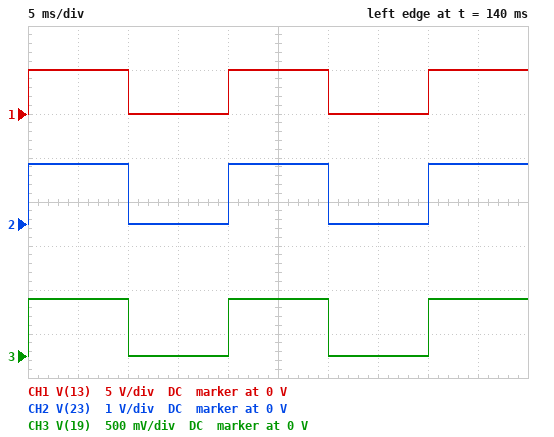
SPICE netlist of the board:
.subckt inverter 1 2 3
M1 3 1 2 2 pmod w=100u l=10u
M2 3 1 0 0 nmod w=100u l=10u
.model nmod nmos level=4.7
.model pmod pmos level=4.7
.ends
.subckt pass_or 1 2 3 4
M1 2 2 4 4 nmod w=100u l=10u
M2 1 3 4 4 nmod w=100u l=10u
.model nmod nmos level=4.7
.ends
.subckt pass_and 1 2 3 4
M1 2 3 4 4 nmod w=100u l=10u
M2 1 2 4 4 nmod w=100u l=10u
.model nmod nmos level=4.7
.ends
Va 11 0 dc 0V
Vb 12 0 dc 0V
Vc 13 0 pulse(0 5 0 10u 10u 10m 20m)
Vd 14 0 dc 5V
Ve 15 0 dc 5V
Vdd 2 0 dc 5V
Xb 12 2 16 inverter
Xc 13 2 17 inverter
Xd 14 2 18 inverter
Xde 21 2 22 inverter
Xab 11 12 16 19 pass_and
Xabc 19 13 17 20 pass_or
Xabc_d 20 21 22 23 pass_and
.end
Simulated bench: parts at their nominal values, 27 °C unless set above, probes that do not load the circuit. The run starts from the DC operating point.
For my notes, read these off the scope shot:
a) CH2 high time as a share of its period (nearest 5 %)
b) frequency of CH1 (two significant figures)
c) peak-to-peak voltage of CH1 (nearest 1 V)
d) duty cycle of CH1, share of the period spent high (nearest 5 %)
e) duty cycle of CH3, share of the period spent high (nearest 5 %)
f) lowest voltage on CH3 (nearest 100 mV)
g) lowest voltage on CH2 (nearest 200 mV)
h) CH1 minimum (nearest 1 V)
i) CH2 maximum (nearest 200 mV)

50 %
50 Hz
5 V
50 %
50 %
0 V
0 V
0 V
1.4 V
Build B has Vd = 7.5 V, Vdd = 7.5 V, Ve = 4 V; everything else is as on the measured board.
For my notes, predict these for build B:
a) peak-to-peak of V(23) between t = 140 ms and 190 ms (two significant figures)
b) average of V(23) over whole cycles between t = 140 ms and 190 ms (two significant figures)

1.3 V
660 mV
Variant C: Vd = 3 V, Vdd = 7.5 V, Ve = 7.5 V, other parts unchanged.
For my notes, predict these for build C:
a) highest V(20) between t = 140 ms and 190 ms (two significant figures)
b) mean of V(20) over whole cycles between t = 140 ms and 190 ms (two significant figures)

1.3 V
660 mV
